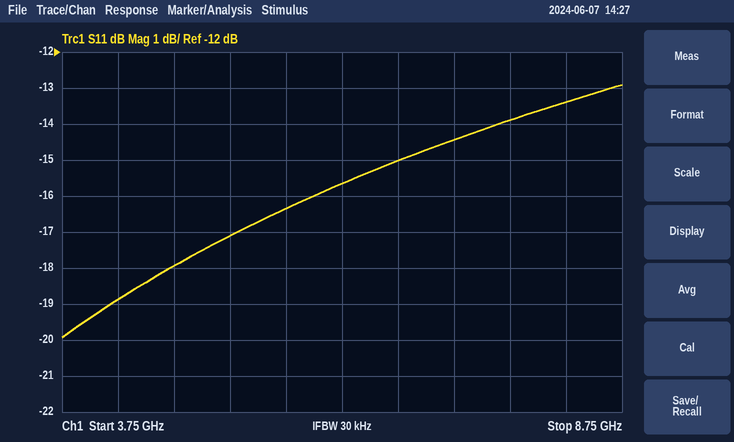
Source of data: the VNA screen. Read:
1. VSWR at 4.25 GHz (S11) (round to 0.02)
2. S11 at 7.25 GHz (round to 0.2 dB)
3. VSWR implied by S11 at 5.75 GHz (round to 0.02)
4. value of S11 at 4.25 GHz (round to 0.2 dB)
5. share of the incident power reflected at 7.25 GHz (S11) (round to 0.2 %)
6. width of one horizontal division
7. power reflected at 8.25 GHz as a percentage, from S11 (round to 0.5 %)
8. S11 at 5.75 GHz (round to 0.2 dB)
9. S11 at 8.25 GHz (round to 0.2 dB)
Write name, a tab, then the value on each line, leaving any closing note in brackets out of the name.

VSWR at 4.25 GHz (S11)	1.26
S11 at 7.25 GHz	-14.4 dB
VSWR implied by S11 at 5.75 GHz	1.36
value of S11 at 4.25 GHz	-18.8 dB
share of the incident power reflected at 7.25 GHz (S11)	3.6 %
width of one horizontal division	500 MHz
power reflected at 8.25 GHz as a percentage, from S11	4.5 %
S11 at 5.75 GHz	-16.4 dB
S11 at 8.25 GHz	-13.4 dB
